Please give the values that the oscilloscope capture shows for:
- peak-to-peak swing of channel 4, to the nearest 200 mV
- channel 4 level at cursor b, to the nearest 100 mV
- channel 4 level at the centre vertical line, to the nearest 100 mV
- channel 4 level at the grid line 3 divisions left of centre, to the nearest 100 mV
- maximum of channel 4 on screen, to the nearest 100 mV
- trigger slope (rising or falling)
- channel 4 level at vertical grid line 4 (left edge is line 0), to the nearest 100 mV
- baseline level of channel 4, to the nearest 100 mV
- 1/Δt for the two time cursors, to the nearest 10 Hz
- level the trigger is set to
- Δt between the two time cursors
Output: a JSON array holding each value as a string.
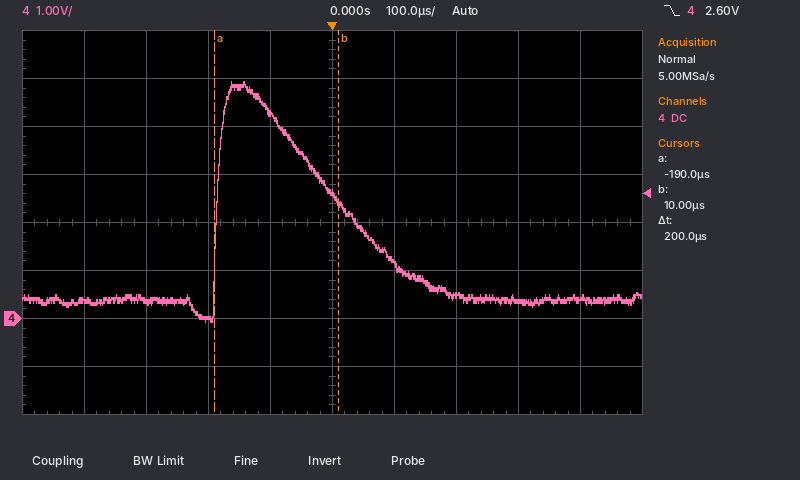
["5.0 V", "2.4 V", "2.6 V", "400 mV", "4.9 V", "falling", "4.3 V", "400 mV", "5.00 kHz", "2.60 V", "200 µs"]
